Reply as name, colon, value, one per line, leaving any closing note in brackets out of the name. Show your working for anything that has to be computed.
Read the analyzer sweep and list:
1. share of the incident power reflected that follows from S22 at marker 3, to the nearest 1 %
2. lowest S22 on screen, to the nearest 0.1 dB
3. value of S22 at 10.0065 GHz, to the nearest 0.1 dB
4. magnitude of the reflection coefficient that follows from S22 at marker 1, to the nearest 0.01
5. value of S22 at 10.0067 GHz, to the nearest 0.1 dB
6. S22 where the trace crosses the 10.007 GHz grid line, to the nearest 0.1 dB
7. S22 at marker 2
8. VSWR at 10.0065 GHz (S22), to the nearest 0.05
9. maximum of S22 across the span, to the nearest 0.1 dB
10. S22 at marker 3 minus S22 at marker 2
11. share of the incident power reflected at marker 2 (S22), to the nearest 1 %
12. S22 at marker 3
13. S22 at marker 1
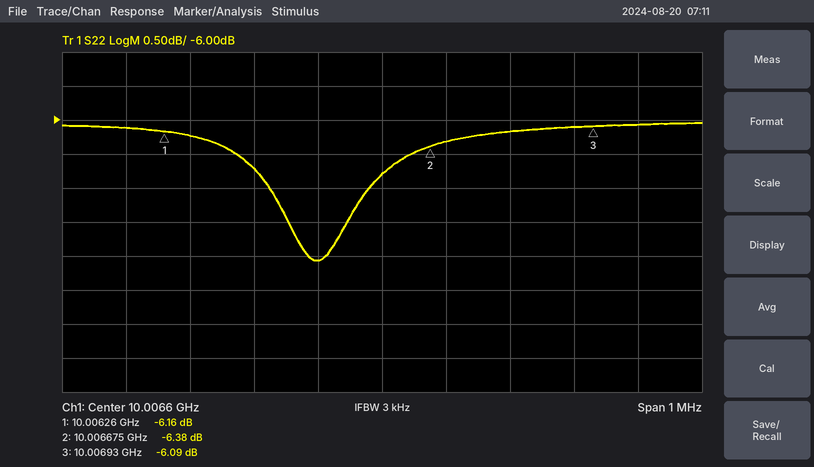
share of the incident power reflected that follows from S22 at marker 3, to the nearest 1 %: 10^(-6.09/10) ≈ 25 %
lowest S22 on screen, to the nearest 0.1 dB: -8.1 dB
value of S22 at 10.0065 GHz, to the nearest 0.1 dB: -8.1 dB
magnitude of the reflection coefficient that follows from S22 at marker 1, to the nearest 0.01: 10^(-6.16/20) ≈ 0.49
value of S22 at 10.0067 GHz, to the nearest 0.1 dB: -6.3 dB
S22 where the trace crosses the 10.007 GHz grid line, to the nearest 0.1 dB: -6.1 dB
S22 at marker 2: -6.38 dB
VSWR at 10.0065 GHz (S22), to the nearest 0.05: |Γ| = 10^(-8.1/20) = 0.3936; VSWR = (1 + 0.3936)/(1 − 0.3936) ≈ 2.30
maximum of S22 across the span, to the nearest 0.1 dB: -6.0 dB
S22 at marker 3 minus S22 at marker 2: -6.09 − (-6.38) = 0.29 dB
share of the incident power reflected at marker 2 (S22), to the nearest 1 %: 10^(-6.38/10) ≈ 23 %
S22 at marker 3: -6.09 dB
S22 at marker 1: -6.16 dB
